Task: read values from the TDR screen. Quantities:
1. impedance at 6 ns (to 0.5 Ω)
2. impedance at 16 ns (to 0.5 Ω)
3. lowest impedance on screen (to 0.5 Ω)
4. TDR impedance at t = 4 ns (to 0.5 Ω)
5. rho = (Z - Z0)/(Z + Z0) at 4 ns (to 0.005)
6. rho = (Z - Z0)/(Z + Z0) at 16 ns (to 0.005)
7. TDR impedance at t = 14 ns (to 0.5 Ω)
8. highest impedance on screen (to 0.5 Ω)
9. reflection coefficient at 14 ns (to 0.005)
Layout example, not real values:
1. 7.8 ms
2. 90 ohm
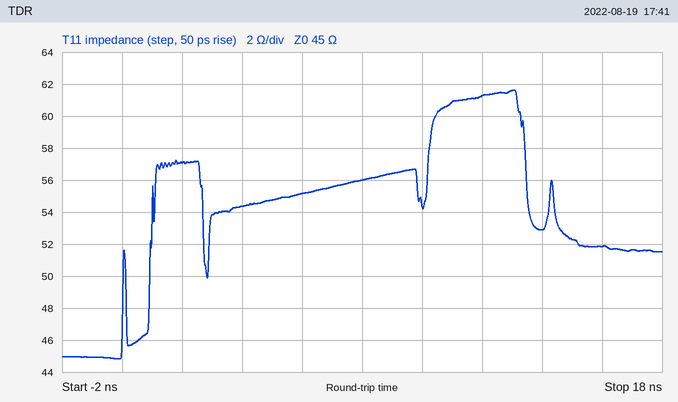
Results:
1. 55.0 Ω
2. 52.0 Ω
3. 45.0 Ω
4. 54.5 Ω
5. +0.095
6. +0.070
7. 53.0 Ω
8. 61.5 Ω
9. +0.080
